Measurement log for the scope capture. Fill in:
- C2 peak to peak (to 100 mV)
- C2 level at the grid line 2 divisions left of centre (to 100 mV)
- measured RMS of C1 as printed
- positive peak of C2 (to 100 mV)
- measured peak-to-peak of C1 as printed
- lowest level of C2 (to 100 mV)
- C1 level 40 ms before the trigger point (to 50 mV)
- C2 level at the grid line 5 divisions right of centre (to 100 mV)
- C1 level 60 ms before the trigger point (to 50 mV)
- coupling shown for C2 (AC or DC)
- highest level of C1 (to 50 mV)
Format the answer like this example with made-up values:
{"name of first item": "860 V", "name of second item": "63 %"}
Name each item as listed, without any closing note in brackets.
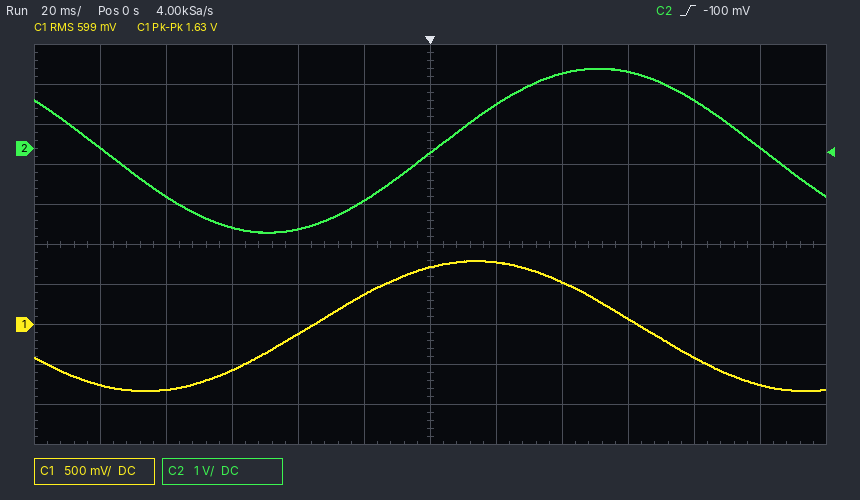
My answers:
{"C2 peak to peak": "4.1 V", "C2 level at the grid line 2 divisions left of centre": "-2.0 V", "measured RMS of C1 as printed": "599 mV", "positive peak of C2": "2.0 V", "measured peak-to-peak of C1 as printed": "1.63 V", "lowest level of C2": "-2.1 V", "C1 level 40 ms before the trigger point": "-100 mV", "C2 level at the grid line 5 divisions right of centre": "0.0 V", "C1 level 60 ms before the trigger point": "-550 mV", "coupling shown for C2": "DC", "highest level of C1": "800 mV"}
